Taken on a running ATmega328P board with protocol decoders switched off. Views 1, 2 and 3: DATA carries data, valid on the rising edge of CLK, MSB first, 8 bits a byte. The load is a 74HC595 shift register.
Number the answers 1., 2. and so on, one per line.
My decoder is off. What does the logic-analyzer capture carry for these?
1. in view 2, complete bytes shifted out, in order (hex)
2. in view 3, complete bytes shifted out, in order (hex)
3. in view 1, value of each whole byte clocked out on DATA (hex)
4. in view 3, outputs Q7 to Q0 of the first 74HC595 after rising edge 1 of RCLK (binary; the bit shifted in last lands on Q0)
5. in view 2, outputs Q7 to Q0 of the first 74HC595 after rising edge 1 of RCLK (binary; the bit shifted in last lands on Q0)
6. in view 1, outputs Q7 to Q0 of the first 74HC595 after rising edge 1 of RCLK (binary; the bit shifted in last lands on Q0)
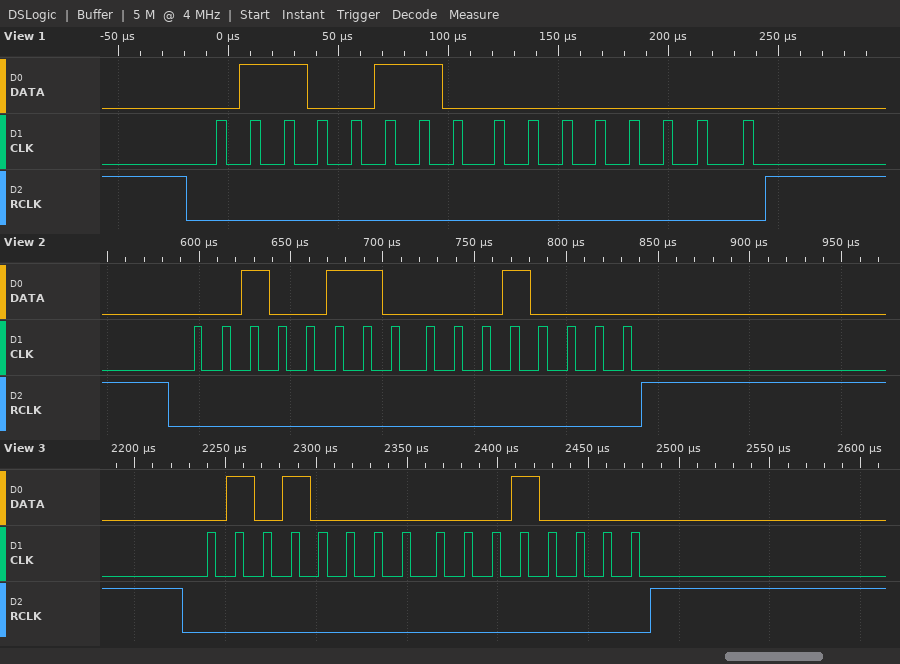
1. 26 10
2. 0x50 0x10
3. 0x66 0x00
4. 00010000
5. 00010000
6. 00000000
